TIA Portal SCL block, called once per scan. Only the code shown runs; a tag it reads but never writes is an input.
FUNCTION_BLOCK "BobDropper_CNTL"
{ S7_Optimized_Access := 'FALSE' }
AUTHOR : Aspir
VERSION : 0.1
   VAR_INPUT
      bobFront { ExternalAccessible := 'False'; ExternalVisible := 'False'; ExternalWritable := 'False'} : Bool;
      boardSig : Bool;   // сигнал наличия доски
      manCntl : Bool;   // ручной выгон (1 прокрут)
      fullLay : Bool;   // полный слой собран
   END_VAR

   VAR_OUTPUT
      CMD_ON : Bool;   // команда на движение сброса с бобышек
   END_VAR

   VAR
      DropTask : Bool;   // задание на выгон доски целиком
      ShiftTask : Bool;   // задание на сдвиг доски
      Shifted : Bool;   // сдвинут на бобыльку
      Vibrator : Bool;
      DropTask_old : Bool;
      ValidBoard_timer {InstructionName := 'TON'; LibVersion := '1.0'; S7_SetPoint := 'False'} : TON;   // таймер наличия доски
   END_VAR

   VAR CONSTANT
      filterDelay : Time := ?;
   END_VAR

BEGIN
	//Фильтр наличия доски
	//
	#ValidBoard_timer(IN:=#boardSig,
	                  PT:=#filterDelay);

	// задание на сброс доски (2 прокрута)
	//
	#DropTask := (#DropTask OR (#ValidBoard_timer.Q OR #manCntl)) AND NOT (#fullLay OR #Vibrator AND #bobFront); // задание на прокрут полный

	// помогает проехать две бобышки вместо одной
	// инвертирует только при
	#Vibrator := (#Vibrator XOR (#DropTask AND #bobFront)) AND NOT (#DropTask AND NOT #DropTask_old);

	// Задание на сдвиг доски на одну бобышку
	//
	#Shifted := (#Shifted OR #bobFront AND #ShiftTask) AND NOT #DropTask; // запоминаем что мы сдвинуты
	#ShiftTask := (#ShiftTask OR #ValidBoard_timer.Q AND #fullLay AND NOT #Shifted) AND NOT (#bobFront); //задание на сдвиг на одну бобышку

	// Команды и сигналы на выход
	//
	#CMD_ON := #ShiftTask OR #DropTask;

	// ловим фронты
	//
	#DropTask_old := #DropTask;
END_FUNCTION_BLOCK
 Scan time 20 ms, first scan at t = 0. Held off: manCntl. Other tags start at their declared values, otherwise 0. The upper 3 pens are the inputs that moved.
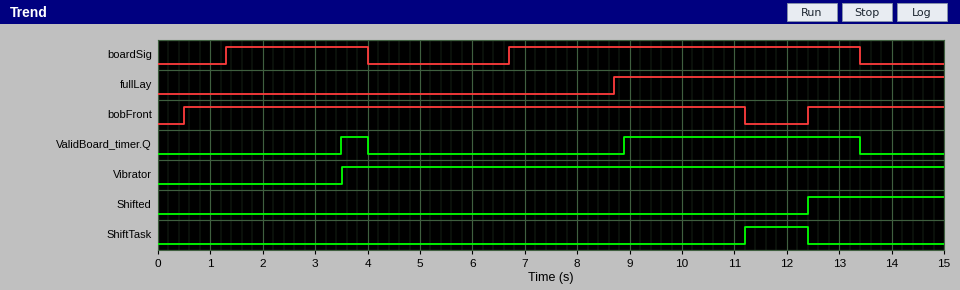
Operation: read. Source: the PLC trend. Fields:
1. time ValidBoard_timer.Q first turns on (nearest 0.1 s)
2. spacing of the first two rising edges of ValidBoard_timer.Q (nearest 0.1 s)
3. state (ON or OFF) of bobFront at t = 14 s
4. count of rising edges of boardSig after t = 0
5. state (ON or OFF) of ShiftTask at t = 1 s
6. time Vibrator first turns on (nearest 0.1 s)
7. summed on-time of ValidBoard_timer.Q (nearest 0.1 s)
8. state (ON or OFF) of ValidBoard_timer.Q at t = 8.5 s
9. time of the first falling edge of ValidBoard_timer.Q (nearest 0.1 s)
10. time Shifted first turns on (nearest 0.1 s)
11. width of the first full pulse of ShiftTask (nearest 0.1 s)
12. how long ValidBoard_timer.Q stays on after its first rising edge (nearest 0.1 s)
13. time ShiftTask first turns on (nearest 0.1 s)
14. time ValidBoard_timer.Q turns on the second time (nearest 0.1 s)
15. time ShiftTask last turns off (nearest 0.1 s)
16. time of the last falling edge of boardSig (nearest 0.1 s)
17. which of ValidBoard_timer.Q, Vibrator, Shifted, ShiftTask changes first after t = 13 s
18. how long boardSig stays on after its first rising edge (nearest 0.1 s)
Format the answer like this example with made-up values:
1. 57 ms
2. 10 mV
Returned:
1. 3.5 s
2. 5.4 s
3. ON
4. 2
5. OFF
6. 3.5 s
7. 5.0 s
8. OFF
9. 4.0 s
10. 12.4 s
11. 1.2 s
12. 0.5 s
13. 11.2 s
14. 8.9 s
15. 12.4 s
16. 13.4 s
17. ValidBoard_timer.Q
18. 2.7 s
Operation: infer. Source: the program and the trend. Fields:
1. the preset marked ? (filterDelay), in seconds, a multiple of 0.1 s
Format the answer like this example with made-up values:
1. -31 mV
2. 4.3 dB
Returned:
1. 2.2 s
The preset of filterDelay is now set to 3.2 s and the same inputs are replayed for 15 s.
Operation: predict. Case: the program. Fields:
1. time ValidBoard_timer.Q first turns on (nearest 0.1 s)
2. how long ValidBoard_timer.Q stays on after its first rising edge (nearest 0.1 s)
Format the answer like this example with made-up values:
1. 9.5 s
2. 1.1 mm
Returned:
1. 9.9 s
2. 3.5 s
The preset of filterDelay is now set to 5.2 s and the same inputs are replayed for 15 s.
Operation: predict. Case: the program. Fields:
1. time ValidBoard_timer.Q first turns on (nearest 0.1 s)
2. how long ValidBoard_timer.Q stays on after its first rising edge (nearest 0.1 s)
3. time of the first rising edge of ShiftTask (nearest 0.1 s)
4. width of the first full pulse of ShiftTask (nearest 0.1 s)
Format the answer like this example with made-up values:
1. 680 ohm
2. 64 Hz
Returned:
1. 11.9 s
2. 1.5 s
3. 11.9 s
4. 0.5 s
